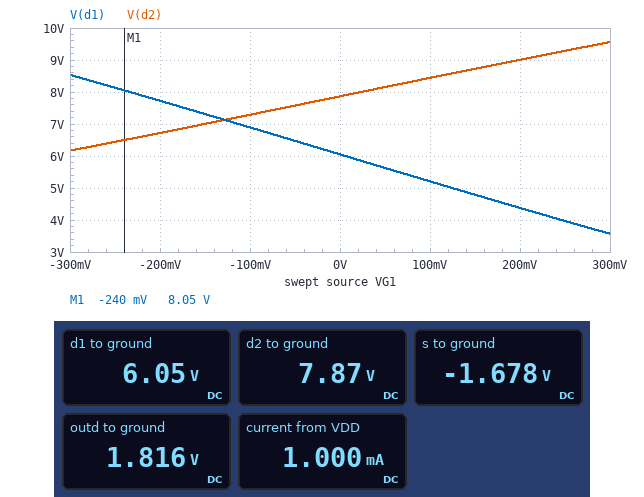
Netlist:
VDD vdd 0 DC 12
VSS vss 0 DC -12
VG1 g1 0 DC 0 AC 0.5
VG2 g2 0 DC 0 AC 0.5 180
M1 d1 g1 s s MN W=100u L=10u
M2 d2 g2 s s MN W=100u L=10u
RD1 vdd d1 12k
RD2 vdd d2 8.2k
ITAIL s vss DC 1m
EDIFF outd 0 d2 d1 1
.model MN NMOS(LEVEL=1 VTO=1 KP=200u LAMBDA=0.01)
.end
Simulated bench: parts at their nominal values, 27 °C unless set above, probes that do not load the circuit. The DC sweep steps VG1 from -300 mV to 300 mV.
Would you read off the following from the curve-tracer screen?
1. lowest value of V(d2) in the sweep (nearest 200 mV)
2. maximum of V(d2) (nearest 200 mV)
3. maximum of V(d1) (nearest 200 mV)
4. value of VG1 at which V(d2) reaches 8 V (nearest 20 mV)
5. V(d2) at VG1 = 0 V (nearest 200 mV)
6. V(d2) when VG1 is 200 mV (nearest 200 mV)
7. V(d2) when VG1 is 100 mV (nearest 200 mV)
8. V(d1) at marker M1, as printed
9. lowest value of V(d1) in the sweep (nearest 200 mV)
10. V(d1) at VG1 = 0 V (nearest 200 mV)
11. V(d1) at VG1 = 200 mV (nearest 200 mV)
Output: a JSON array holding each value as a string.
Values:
["6.2 V", "9.6 V", "8.6 V", "20 mV", "7.8 V", "9.0 V", "8.4 V", "8.05 V", "3.6 V", "6.0 V", "4.4 V"]
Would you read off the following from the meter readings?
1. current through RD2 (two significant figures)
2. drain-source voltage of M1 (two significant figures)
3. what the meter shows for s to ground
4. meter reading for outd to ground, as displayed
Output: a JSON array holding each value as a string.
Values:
["500 µA", "7.7 V", "-1.678 V", "1.816 V"]
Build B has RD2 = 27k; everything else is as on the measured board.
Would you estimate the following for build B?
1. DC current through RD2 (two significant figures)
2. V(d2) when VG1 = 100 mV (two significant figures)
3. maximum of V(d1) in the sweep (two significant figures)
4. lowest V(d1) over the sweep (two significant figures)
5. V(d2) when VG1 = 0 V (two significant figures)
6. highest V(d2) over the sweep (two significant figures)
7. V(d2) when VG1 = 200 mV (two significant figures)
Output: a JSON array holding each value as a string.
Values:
["480 µA", "720 mV", "6.1 V", "3.5 V", "-1.0 V", "4.2 V", "2.5 V"]
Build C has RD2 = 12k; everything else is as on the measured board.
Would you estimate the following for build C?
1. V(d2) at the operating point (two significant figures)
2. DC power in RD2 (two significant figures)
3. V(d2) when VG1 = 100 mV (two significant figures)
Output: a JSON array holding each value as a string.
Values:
["6.0 V", "3.0 mW", "6.8 V"]
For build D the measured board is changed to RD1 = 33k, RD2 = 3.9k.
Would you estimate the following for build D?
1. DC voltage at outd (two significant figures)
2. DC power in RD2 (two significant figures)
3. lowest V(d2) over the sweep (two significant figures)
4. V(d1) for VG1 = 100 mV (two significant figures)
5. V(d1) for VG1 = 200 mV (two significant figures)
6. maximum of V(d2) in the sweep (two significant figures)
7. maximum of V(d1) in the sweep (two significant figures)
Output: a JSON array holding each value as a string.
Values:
["11 V", "1.4 mW", "9.2 V", "-1.4 V", "-1.5 V", "9.7 V", "3.0 V"]
